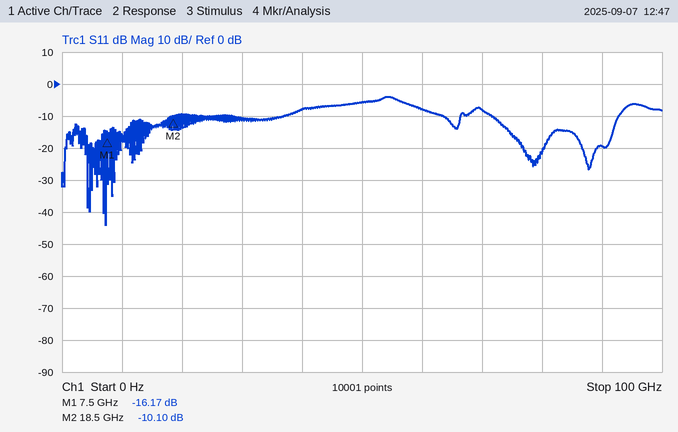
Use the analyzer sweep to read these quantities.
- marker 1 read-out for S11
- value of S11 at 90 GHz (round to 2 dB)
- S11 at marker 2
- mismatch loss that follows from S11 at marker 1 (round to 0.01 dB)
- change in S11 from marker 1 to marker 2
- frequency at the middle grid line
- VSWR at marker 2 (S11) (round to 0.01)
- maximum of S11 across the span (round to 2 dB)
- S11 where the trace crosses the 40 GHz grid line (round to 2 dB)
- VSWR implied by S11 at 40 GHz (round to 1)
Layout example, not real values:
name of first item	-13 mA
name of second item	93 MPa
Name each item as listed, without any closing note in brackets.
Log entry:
marker 1 read-out for S11	-16.17 dB
value of S11 at 90 GHz	-20 dB
S11 at marker 2	-10.10 dB
mismatch loss that follows from S11 at marker 1	0.11 dB
change in S11 from marker 1 to marker 2	6.07 dB
frequency at the middle grid line	50 GHz
VSWR at marker 2 (S11)	1.91
maximum of S11 across the span	-4 dB
S11 where the trace crosses the 40 GHz grid line	-8 dB
VSWR implied by S11 at 40 GHz	2
